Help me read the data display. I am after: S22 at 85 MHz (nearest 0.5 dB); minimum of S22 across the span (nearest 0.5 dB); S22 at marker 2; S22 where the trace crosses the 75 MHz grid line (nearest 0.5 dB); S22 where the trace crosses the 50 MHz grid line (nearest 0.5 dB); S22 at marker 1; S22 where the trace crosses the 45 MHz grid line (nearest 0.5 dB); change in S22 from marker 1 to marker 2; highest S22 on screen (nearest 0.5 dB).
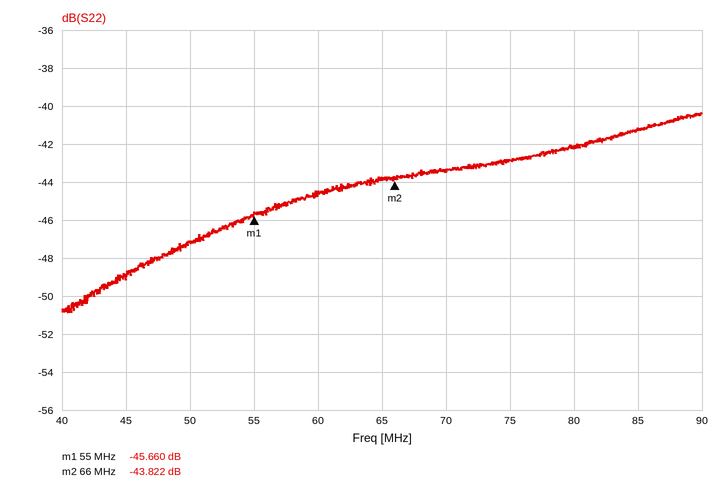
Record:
-41.0 dB
-51.0 dB
-43.822 dB
-43.0 dB
-47.0 dB
-45.660 dB
-49.0 dB
1.838 dB
-40.5 dB
